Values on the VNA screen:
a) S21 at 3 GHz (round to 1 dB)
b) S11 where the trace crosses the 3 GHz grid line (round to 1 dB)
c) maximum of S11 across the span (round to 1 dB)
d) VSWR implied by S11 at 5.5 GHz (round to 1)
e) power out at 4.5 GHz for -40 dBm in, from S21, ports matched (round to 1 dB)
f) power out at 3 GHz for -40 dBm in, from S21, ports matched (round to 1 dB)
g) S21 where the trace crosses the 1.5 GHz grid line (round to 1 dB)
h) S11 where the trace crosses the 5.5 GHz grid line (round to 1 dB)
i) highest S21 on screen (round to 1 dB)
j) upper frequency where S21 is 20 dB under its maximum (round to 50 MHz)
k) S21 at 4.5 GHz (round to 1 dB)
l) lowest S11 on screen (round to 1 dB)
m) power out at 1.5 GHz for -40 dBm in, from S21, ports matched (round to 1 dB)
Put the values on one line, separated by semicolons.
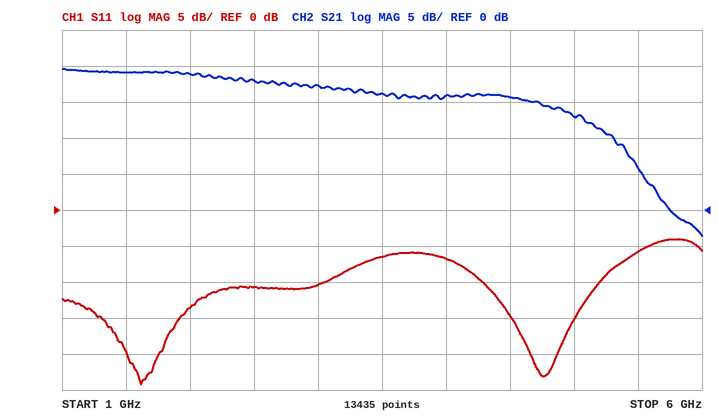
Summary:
17 dB; -10 dB; -4 dB; 3; -24 dBm; -23 dBm; 19 dB; -6 dB; 20 dB; 5.75 GHz; 16 dB; -24 dB; -21 dBm
